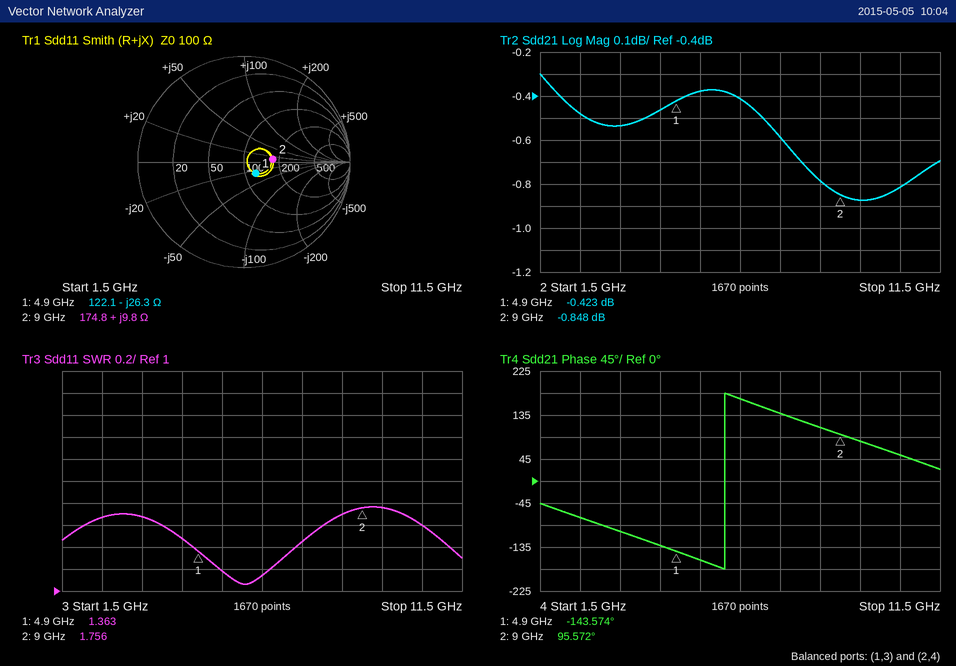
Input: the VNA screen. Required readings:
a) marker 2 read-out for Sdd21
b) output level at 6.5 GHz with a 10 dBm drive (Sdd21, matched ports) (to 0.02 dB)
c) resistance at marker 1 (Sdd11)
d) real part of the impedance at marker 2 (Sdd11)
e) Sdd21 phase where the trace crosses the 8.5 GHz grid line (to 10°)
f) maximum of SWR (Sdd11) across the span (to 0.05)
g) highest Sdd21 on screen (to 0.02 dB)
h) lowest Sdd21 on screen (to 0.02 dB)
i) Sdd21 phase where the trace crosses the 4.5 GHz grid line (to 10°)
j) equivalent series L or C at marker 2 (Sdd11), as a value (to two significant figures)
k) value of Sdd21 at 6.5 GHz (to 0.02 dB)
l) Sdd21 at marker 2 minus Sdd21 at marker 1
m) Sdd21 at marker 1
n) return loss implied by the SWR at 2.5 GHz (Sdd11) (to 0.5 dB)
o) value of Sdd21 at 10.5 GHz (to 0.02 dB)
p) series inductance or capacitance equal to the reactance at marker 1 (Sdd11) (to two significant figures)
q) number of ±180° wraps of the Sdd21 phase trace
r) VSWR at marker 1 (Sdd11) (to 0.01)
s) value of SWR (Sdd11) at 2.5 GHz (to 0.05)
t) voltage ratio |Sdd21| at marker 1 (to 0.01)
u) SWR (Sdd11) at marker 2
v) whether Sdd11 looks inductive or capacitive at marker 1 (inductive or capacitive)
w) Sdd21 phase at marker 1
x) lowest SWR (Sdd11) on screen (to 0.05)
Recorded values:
-0.848 dB
9.58 dBm
122.1 Ω
174.8 Ω
110°
1.75
-0.30 dB
-0.88 dB
-130°
170 pH
-0.42 dB
-0.425 dB
-0.423 dB
12.0 dB
-0.82 dB
1.2 pF
1
1.36
1.65
0.95
1.756
capacitive
-143.574°
1.05
